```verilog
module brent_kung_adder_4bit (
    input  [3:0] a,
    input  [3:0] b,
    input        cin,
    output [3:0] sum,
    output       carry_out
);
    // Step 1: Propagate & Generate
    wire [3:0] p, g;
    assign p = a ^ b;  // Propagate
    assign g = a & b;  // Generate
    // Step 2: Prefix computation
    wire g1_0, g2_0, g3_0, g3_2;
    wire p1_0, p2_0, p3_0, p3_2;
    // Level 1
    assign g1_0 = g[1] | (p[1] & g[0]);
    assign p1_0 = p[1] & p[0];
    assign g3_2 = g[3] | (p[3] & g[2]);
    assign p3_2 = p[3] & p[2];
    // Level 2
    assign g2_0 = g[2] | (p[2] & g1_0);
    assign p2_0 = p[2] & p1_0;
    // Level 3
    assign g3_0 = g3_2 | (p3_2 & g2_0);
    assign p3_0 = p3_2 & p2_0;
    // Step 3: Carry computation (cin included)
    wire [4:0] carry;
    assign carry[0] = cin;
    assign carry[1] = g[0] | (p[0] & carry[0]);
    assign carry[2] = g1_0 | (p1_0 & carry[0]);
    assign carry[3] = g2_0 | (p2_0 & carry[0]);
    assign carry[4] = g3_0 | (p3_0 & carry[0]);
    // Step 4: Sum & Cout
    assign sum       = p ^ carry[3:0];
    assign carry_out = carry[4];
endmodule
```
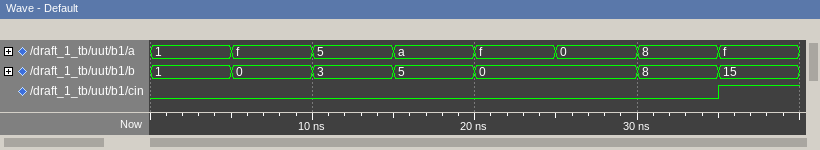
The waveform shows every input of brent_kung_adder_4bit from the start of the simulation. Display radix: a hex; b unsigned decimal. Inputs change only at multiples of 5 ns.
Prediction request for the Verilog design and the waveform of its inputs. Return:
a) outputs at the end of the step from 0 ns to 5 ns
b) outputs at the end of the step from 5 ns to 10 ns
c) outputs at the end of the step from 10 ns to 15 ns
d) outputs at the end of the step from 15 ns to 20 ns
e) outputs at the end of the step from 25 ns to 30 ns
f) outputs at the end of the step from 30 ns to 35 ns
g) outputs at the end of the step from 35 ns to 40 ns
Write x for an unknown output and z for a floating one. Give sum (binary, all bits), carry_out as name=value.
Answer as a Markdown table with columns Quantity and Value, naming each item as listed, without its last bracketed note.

| Quantity | Value |
|---|---|
| outputs at the end of the step from 0 ns to 5 ns | sum=0010, carry_out=0 |
| outputs at the end of the step from 5 ns to 10 ns | sum=1111, carry_out=0 |
| outputs at the end of the step from 10 ns to 15 ns | sum=1000, carry_out=0 |
| outputs at the end of the step from 15 ns to 20 ns | sum=1111, carry_out=0 |
| outputs at the end of the step from 25 ns to 30 ns | sum=0000, carry_out=0 |
| outputs at the end of the step from 30 ns to 35 ns | sum=0000, carry_out=1 |
| outputs at the end of the step from 35 ns to 40 ns | sum=1111, carry_out=1 |
